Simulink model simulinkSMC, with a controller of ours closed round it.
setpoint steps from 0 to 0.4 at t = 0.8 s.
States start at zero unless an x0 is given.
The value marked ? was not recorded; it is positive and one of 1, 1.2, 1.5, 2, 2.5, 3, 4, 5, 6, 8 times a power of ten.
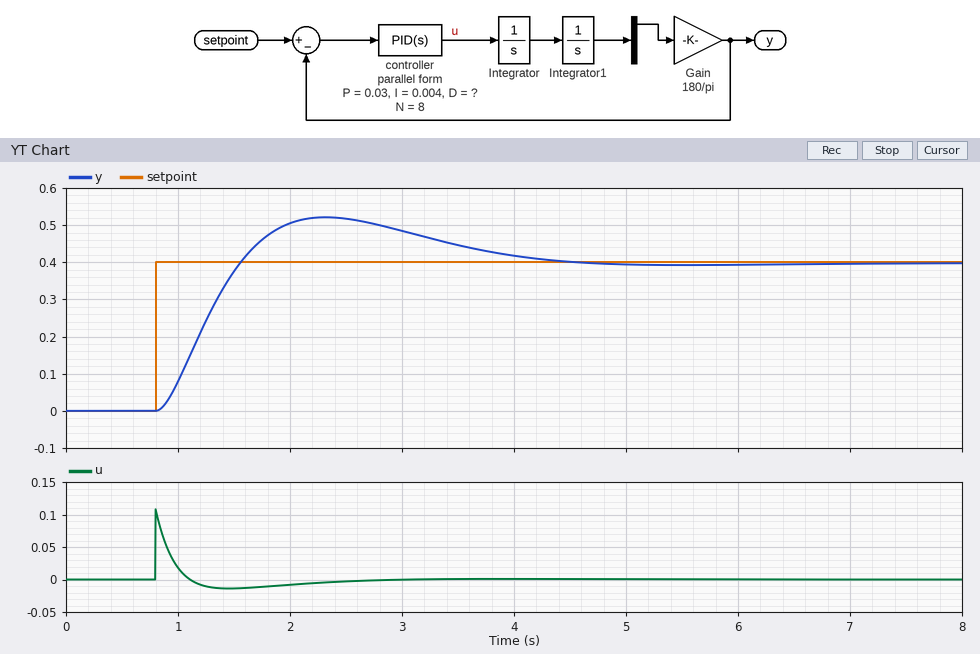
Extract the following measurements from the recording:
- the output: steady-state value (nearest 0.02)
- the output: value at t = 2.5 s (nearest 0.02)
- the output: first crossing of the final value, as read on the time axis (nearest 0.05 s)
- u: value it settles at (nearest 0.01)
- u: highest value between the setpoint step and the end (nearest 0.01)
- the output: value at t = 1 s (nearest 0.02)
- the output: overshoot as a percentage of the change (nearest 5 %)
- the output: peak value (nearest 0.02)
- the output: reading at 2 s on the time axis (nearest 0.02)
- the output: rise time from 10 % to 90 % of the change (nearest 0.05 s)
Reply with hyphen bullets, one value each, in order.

- 0.40
- 0.52
- 1.55 s
- 0.00
- 0.11
- 0.08
- 30 %
- 0.52
- 0.50
- 0.55 s
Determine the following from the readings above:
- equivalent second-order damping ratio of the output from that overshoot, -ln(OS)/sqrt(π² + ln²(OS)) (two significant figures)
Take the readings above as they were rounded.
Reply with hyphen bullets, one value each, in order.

- 0.36
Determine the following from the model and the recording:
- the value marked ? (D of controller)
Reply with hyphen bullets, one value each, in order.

- 0.03
